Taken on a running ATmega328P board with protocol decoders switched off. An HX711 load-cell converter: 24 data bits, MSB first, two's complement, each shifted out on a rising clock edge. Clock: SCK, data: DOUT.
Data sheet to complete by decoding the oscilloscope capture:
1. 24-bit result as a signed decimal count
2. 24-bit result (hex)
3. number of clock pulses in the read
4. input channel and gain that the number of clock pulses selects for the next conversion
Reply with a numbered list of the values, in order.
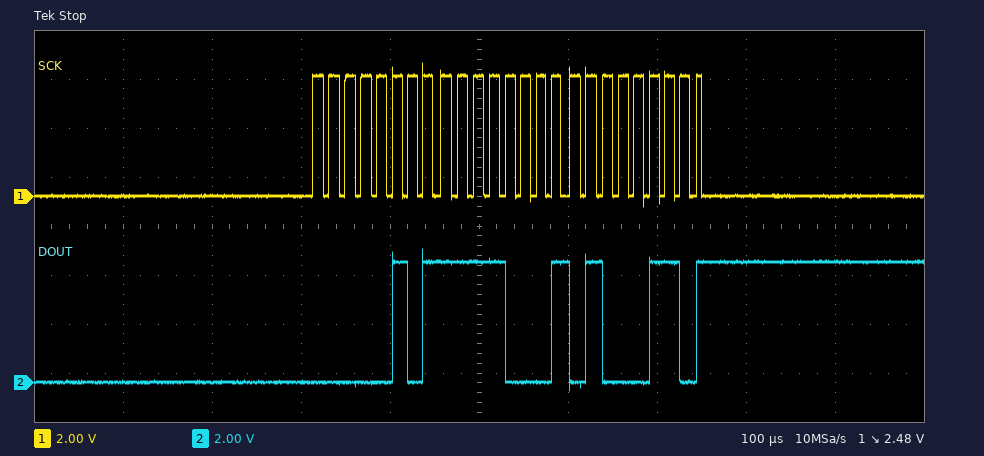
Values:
1. 389446
2. 0x05F146
3. 25
4. channel A, gain 128
